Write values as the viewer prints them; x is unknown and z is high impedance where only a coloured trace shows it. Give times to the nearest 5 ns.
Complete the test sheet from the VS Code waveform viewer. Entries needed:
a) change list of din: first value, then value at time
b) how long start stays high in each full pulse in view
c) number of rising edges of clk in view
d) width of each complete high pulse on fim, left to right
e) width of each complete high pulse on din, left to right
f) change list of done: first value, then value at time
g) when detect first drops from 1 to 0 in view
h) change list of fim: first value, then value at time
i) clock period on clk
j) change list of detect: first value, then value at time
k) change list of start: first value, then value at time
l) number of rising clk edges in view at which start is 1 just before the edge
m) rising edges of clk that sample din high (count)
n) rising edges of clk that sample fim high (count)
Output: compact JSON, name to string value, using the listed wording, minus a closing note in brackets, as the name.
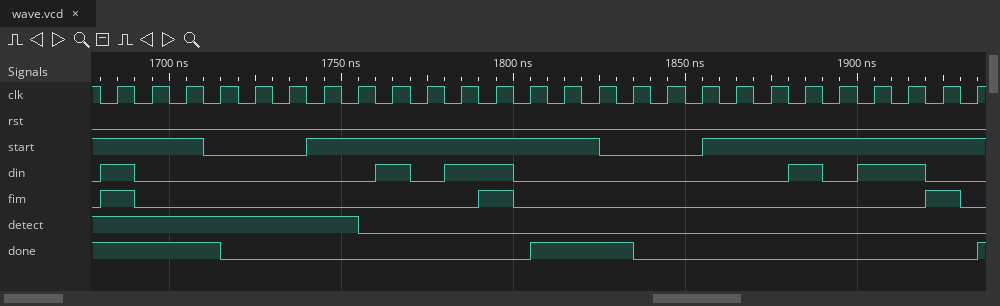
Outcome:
{"change list of din: first value, then value at time": "0, 1 at 1680 ns, 0 at 1690 ns, 1 at 1760 ns, 0 at 1770 ns, 1 at 1780 ns, 0 at 1800 ns, 1 at 1880 ns, 0 at 1890 ns, 1 at 1900 ns, 0 at 1920 ns", "how long start stays high in each full pulse in view": "85 ns", "number of rising edges of clk in view": "26", "width of each complete high pulse on fim, left to right": "10 ns, 10 ns, 10 ns", "width of each complete high pulse on din, left to right": "10 ns, 10 ns, 20 ns, 10 ns, 20 ns", "change list of done: first value, then value at time": "1, 0 at 1715 ns, 1 at 1805 ns, 0 at 1835 ns, 1 at 1935 ns", "when detect first drops from 1 to 0 in view": "1755 ns", "change list of fim: first value, then value at time": "0, 1 at 1680 ns, 0 at 1690 ns, 1 at 1790 ns, 0 at 1800 ns, 1 at 1920 ns, 0 at 1930 ns", "clock period on clk": "10 ns", "change list of detect: first value, then value at time": "1, 0 at 1755 ns", "change list of start: first value, then value at time": "1, 0 at 1710 ns, 1 at 1740 ns, 0 at 1825 ns, 1 at 1855 ns", "number of rising clk edges in view at which start is 1 just before the edge": "20", "rising edges of clk that sample din high": "7", "rising edges of clk that sample fim high": "3"}
